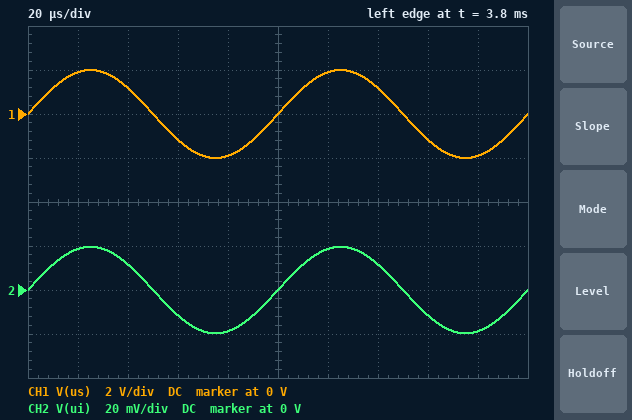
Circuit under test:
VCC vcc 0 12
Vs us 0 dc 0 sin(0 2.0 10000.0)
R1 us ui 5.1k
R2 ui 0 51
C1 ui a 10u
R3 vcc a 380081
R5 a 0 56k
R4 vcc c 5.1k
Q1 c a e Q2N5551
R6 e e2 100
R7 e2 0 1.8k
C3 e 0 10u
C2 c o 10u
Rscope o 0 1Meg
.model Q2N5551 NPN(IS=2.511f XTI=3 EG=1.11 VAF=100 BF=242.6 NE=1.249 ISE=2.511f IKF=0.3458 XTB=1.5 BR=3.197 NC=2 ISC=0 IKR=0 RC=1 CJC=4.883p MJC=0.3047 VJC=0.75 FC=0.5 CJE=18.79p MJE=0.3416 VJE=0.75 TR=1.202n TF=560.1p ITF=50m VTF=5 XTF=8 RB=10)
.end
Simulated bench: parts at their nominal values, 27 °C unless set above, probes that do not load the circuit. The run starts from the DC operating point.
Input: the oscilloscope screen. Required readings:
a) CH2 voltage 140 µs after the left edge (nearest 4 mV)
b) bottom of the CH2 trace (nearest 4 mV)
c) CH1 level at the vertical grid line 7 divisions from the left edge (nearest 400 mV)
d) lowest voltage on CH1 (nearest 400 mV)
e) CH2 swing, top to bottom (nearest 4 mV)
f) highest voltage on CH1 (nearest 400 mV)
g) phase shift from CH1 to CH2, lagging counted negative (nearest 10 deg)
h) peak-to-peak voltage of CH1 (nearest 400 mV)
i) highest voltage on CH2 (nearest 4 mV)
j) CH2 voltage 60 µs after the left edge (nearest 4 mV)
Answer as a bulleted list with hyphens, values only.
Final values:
- 12 mV
- -20 mV
- 1.2 V
- -2.0 V
- 40 mV
- 2.0 V
- 0 deg
- 4.0 V
- 20 mV
- -12 mV
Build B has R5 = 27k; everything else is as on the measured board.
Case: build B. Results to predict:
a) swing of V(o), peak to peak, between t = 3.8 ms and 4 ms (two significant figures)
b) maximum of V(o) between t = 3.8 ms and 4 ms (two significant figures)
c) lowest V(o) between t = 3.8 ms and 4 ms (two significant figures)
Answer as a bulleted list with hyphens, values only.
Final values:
- 610 mV
- 230 mV
- -380 mV
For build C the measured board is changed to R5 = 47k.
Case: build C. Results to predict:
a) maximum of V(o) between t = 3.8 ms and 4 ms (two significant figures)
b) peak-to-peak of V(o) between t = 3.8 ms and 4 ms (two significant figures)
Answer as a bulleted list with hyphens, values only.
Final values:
- 850 mV
- 2.1 V
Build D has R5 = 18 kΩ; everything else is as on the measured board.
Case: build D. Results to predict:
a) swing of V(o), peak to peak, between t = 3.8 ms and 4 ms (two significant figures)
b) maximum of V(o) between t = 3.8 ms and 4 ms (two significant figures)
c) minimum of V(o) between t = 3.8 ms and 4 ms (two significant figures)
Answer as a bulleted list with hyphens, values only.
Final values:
- 24 mV
- 7.7 mV
- -16 mV
